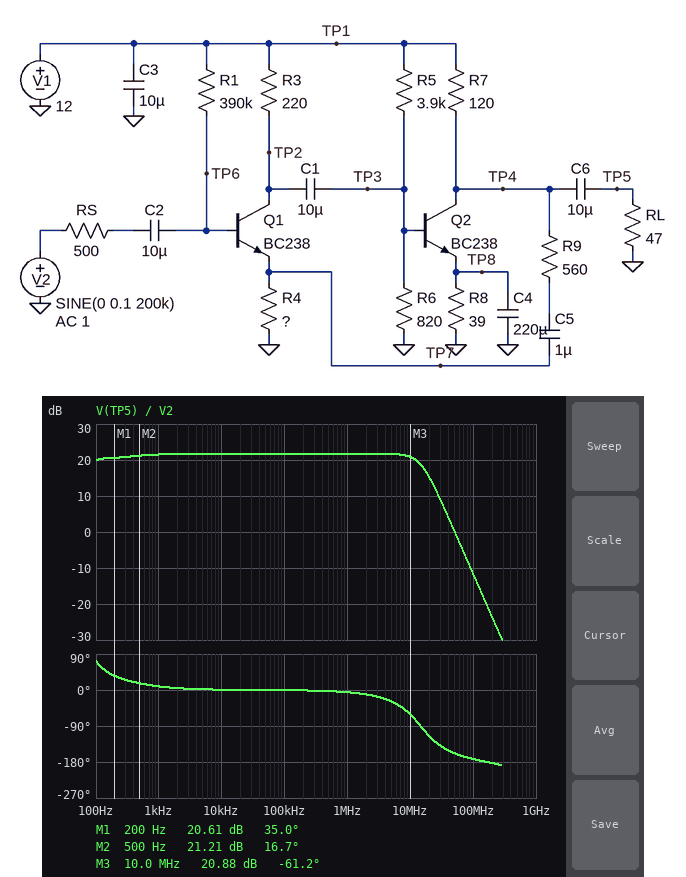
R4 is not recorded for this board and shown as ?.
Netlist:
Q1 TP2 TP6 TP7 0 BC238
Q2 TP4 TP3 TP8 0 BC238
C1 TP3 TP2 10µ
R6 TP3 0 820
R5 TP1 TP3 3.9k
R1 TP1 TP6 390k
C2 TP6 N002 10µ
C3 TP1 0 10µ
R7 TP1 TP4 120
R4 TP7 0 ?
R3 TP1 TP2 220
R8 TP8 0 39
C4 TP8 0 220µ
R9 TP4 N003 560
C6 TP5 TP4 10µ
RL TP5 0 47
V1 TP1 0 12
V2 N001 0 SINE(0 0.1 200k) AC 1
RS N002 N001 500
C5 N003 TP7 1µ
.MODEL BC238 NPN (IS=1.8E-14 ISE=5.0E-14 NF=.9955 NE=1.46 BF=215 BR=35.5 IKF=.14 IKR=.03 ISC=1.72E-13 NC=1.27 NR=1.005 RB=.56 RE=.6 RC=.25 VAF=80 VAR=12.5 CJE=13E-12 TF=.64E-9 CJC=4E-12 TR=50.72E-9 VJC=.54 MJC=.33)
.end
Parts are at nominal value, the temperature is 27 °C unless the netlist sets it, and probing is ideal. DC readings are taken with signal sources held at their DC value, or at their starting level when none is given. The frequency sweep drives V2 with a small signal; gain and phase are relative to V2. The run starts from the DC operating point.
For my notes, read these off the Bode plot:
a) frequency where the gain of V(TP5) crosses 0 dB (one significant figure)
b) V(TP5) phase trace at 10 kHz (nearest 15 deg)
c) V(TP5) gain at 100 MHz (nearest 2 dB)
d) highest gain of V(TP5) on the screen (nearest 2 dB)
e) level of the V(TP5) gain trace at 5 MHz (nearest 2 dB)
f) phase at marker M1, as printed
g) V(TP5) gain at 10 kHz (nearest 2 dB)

50 MHz
0 deg
-12 dB
22 dB
22 dB
35.0 deg
22 dB
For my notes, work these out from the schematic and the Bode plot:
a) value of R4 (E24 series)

36 Ω
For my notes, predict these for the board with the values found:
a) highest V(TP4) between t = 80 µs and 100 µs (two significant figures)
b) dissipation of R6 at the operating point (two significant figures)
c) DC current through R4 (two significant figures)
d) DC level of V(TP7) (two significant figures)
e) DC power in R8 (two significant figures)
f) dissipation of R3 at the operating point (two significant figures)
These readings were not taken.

9.3 V
4.7 mW
5.6 mA
200 mV
38 mW
6.8 mW
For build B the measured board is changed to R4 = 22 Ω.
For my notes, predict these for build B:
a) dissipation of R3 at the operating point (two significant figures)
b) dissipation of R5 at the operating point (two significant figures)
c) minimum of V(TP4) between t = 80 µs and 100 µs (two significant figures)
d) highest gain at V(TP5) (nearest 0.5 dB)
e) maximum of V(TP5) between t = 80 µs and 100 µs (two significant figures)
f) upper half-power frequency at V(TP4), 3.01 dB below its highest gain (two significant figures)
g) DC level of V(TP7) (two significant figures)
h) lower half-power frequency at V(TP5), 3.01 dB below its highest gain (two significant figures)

6.9 mW
26 mW
6.4 V
25.5 dB
1.0 V
160 Hz
120 mV
85 Hz
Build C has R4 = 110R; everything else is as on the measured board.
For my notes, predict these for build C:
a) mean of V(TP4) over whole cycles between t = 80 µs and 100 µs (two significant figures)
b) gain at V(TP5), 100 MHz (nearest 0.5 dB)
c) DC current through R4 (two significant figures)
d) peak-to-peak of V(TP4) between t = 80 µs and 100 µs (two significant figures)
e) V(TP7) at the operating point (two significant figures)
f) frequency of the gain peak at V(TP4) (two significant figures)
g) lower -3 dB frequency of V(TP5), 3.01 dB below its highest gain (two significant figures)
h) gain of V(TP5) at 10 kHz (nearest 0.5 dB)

8.3 V
-13.5 dB
5.4 mA
920 mV
590 mV
77 Hz
84 Hz
13.5 dB
